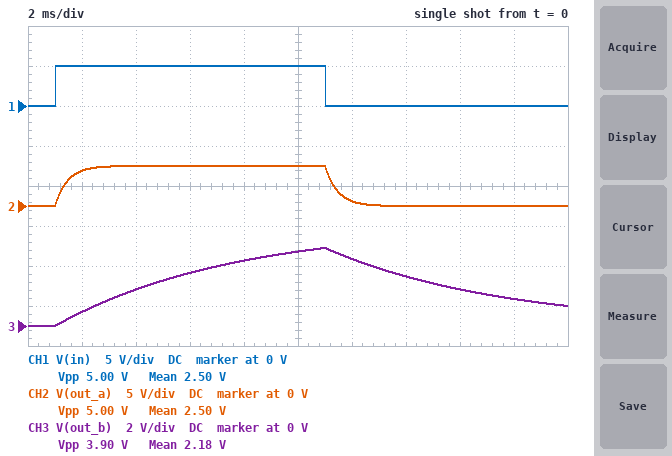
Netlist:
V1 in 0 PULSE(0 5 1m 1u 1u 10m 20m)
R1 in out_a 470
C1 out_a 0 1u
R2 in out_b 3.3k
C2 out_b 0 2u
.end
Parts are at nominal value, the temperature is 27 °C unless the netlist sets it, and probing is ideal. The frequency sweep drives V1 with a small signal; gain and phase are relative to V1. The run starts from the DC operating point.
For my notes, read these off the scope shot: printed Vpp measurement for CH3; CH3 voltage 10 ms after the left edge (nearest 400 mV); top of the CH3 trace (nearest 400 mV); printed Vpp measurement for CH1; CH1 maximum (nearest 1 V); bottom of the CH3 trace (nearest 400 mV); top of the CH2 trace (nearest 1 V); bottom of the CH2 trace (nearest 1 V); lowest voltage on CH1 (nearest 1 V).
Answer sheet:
3.90 V
3.6 V
4.0 V
5.00 V
5 V
0 V
5 V
0 V
0 V
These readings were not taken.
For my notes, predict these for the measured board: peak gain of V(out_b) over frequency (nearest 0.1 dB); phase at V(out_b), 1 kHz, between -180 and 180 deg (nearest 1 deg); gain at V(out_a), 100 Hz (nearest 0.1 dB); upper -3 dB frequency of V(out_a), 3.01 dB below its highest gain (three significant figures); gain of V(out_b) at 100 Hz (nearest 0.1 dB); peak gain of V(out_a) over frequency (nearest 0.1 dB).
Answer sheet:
0 dB
-89 deg
-0.4 dB
339 Hz
-12.6 dB
0 dB
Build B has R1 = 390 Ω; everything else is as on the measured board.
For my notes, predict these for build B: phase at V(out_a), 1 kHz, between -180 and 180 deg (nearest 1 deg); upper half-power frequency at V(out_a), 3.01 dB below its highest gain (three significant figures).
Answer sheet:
-68 deg
408 Hz
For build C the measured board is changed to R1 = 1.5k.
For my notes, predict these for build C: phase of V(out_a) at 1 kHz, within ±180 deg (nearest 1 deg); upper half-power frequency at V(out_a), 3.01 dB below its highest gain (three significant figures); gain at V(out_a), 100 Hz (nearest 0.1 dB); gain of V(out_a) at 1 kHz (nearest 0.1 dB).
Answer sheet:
-84 deg
106 Hz
-2.8 dB
-19.5 dB
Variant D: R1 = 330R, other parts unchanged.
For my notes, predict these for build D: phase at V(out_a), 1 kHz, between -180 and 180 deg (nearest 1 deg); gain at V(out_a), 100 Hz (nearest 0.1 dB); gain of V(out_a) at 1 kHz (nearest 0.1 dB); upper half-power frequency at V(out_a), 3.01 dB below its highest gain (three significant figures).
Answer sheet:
-64 deg
-0.2 dB
-7.2 dB
482 Hz
